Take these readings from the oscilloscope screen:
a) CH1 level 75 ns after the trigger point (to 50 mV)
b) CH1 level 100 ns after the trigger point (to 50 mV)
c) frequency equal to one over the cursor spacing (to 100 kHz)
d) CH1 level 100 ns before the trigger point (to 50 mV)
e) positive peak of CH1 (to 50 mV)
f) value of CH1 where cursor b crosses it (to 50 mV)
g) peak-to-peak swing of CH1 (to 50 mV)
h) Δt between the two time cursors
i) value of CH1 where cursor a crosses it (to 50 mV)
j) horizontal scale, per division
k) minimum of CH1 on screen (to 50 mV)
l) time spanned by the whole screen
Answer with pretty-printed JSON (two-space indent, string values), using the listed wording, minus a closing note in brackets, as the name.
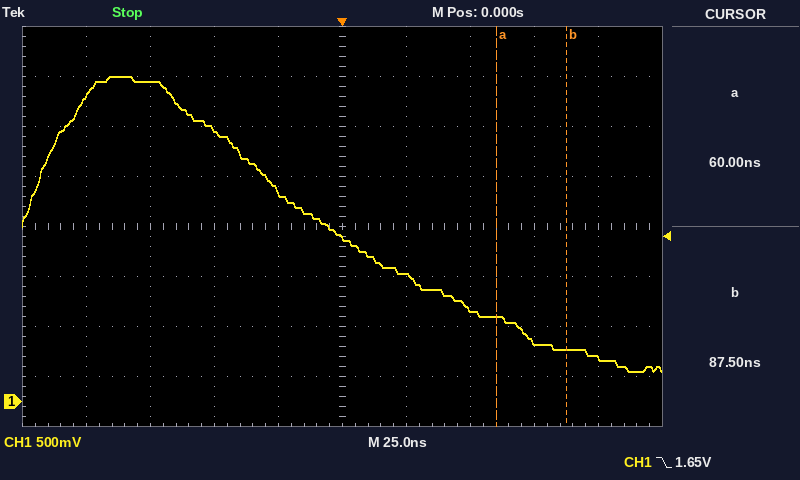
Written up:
{
  "CH1 level 75 ns after the trigger point": "600 mV",
  "CH1 level 100 ns after the trigger point": "450 mV",
  "frequency equal to one over the cursor spacing": "36.4 MHz",
  "CH1 level 100 ns before the trigger point": "3.05 V",
  "positive peak of CH1": "3.25 V",
  "value of CH1 where cursor b crosses it": "500 mV",
  "peak-to-peak swing of CH1": "2.95 V",
  "Δt between the two time cursors": "27.5 ns",
  "value of CH1 where cursor a crosses it": "850 mV",
  "horizontal scale, per division": "25 ns",
  "minimum of CH1 on screen": "300 mV",
  "time spanned by the whole screen": "250 ns"
}
